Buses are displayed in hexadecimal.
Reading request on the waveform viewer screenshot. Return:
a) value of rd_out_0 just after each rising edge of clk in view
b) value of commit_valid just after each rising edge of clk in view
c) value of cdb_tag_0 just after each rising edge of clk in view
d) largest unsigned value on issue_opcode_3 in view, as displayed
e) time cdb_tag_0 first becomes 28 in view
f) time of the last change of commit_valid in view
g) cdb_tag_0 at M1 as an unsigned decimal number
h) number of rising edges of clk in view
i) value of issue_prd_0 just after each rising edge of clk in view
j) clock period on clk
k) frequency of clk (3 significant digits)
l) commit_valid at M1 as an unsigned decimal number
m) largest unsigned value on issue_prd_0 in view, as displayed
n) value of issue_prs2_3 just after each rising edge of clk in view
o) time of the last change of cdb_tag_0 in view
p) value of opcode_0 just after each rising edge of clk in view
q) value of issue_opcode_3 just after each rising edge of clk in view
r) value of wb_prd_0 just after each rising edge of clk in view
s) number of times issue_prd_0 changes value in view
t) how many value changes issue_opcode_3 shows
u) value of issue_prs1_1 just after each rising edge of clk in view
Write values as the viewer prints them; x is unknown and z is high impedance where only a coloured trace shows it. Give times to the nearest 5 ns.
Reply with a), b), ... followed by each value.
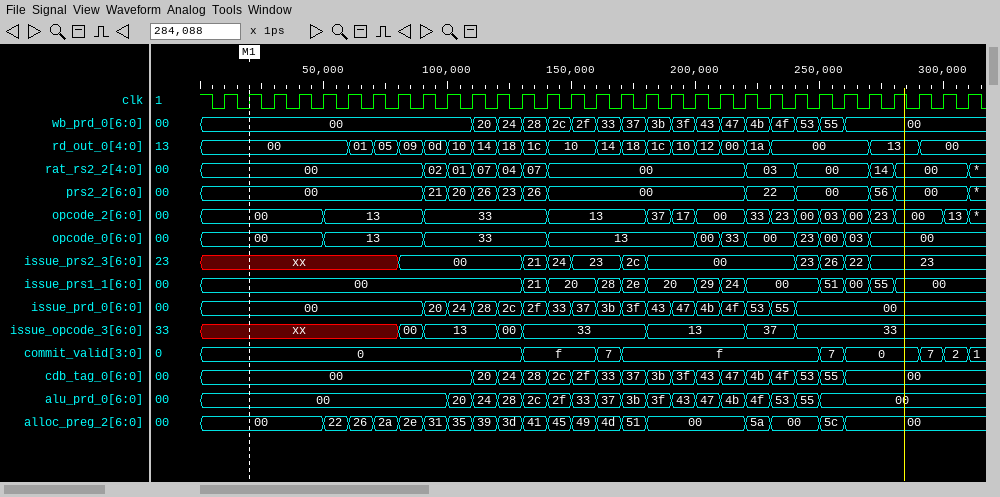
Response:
a) 00, 00, 00, 00, 00, 01, 05, 09, 0d, 10, 14, 18, 1c, 10, 10, 14, 18, 1c, 10, 12, 00, 1a, 00, 00, 00, 00, 13, 13, 00, 00, 00
b) 0, 0, 0, 0, 0, 0, 0, 0, 0, 0, 0, 0, f, f, f, 7, f, f, f, f, f, f, f, f, 7, 0, 0, 0, 7, 2, 1
c) 00, 00, 00, 00, 00, 00, 00, 00, 00, 00, 20, 24, 28, 2c, 2f, 33, 37, 3b, 3f, 43, 47, 4b, 4f, 53, 55, 00, 00, 00, 00, 00, 00
d) 37
e) 130 ns
f) 310 ns
g) 0
h) 31
i) 00, 00, 00, 00, 00, 00, 00, 00, 20, 24, 28, 2c, 2f, 33, 37, 3b, 3f, 43, 47, 4b, 4f, 53, 55, 00, 00, 00, 00, 00, 00, 00, 00
j) 10 ns
k) 100 MHz
l) 0
m) 55
n) xx, xx, xx, xx, xx, xx, xx, 00, 00, 00, 00, 00, 21, 24, 23, 23, 2c, 00, 00, 00, 00, 00, 00, 23, 26, 22, 23, 23, 23, 23, 23
o) 260 ns
p) 00, 00, 00, 00, 13, 13, 13, 13, 33, 33, 33, 33, 33, 13, 13, 13, 13, 13, 13, 00, 33, 00, 00, 23, 00, 03, 00, 00, 00, 00, 00
q) xx, xx, xx, xx, xx, xx, xx, 00, 13, 13, 13, 00, 33, 33, 33, 33, 33, 13, 13, 13, 13, 37, 37, 33, 33, 33, 33, 33, 33, 33, 33
r) 00, 00, 00, 00, 00, 00, 00, 00, 00, 00, 20, 24, 28, 2c, 2f, 33, 37, 3b, 3f, 43, 47, 4b, 4f, 53, 55, 00, 00, 00, 00, 00, 00
s) 16
t) 7
u) 00, 00, 00, 00, 00, 00, 00, 00, 00, 00, 00, 00, 21, 20, 20, 28, 2e, 20, 20, 29, 24, 00, 00, 00, 51, 00, 55, 00, 00, 00, 00
